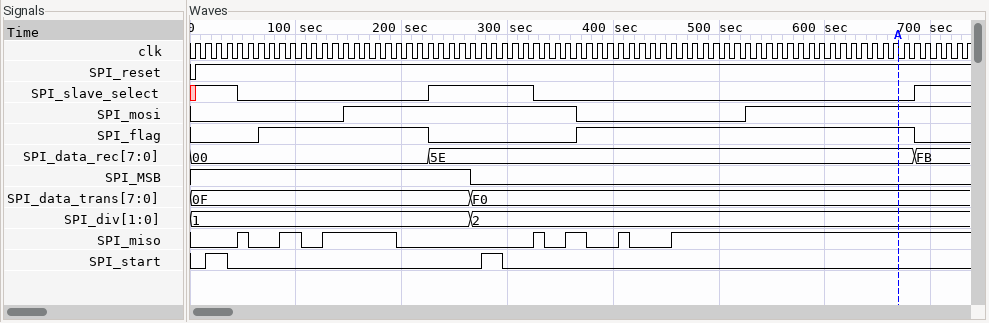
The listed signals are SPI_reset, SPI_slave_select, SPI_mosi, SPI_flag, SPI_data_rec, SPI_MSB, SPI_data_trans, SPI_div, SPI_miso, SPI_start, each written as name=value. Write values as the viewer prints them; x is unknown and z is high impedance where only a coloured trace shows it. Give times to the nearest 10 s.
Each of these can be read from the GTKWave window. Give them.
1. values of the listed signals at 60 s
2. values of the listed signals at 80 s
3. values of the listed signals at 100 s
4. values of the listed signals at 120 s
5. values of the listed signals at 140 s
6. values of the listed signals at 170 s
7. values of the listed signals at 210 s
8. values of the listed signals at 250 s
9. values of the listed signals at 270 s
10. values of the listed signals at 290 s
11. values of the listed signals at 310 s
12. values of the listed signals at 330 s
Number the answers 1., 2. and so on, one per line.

1. SPI_reset=1, SPI_slave_select=0, SPI_mosi=0, SPI_flag=0, SPI_data_rec=00, SPI_MSB=1, SPI_data_trans=0F, SPI_div=1, SPI_miso=0, SPI_start=0
2. SPI_reset=1, SPI_slave_select=0, SPI_mosi=0, SPI_flag=1, SPI_data_rec=00, SPI_MSB=1, SPI_data_trans=0F, SPI_div=1, SPI_miso=0, SPI_start=0
3. SPI_reset=1, SPI_slave_select=0, SPI_mosi=0, SPI_flag=1, SPI_data_rec=00, SPI_MSB=1, SPI_data_trans=0F, SPI_div=1, SPI_miso=1, SPI_start=0
4. SPI_reset=1, SPI_slave_select=0, SPI_mosi=0, SPI_flag=1, SPI_data_rec=00, SPI_MSB=1, SPI_data_trans=0F, SPI_div=1, SPI_miso=0, SPI_start=0
5. SPI_reset=1, SPI_slave_select=0, SPI_mosi=0, SPI_flag=1, SPI_data_rec=00, SPI_MSB=1, SPI_data_trans=0F, SPI_div=1, SPI_miso=1, SPI_start=0
6. SPI_reset=1, SPI_slave_select=0, SPI_mosi=1, SPI_flag=1, SPI_data_rec=00, SPI_MSB=1, SPI_data_trans=0F, SPI_div=1, SPI_miso=1, SPI_start=0
7. SPI_reset=1, SPI_slave_select=0, SPI_mosi=1, SPI_flag=1, SPI_data_rec=00, SPI_MSB=1, SPI_data_trans=0F, SPI_div=1, SPI_miso=0, SPI_start=0
8. SPI_reset=1, SPI_slave_select=1, SPI_mosi=1, SPI_flag=0, SPI_data_rec=5E, SPI_MSB=1, SPI_data_trans=0F, SPI_div=1, SPI_miso=0, SPI_start=0
9. SPI_reset=1, SPI_slave_select=1, SPI_mosi=1, SPI_flag=0, SPI_data_rec=5E, SPI_MSB=0, SPI_data_trans=F0, SPI_div=2, SPI_miso=0, SPI_start=0
10. SPI_reset=1, SPI_slave_select=1, SPI_mosi=1, SPI_flag=0, SPI_data_rec=5E, SPI_MSB=0, SPI_data_trans=F0, SPI_div=2, SPI_miso=0, SPI_start=1
11. SPI_reset=1, SPI_slave_select=1, SPI_mosi=1, SPI_flag=0, SPI_data_rec=5E, SPI_MSB=0, SPI_data_trans=F0, SPI_div=2, SPI_miso=0, SPI_start=0
12. SPI_reset=1, SPI_slave_select=0, SPI_mosi=1, SPI_flag=0, SPI_data_rec=5E, SPI_MSB=0, SPI_data_trans=F0, SPI_div=2, SPI_miso=1, SPI_start=0
